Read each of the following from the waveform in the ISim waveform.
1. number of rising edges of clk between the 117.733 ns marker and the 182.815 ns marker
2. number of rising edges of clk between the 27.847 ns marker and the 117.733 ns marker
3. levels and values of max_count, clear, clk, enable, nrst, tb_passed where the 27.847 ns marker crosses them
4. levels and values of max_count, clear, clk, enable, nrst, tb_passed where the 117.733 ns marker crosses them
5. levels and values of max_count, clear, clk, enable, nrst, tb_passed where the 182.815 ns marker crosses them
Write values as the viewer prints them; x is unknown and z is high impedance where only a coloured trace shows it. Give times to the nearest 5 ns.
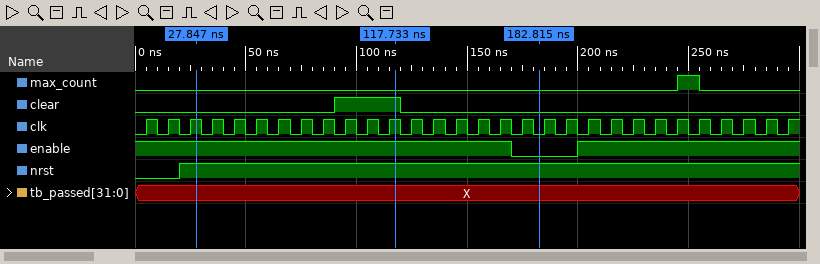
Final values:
6
9
max_count=0, clear=0, clk=1, enable=1, nrst=1, tb_passed=X
max_count=0, clear=1, clk=1, enable=1, nrst=1, tb_passed=X
max_count=0, clear=0, clk=0, enable=0, nrst=1, tb_passed=X
